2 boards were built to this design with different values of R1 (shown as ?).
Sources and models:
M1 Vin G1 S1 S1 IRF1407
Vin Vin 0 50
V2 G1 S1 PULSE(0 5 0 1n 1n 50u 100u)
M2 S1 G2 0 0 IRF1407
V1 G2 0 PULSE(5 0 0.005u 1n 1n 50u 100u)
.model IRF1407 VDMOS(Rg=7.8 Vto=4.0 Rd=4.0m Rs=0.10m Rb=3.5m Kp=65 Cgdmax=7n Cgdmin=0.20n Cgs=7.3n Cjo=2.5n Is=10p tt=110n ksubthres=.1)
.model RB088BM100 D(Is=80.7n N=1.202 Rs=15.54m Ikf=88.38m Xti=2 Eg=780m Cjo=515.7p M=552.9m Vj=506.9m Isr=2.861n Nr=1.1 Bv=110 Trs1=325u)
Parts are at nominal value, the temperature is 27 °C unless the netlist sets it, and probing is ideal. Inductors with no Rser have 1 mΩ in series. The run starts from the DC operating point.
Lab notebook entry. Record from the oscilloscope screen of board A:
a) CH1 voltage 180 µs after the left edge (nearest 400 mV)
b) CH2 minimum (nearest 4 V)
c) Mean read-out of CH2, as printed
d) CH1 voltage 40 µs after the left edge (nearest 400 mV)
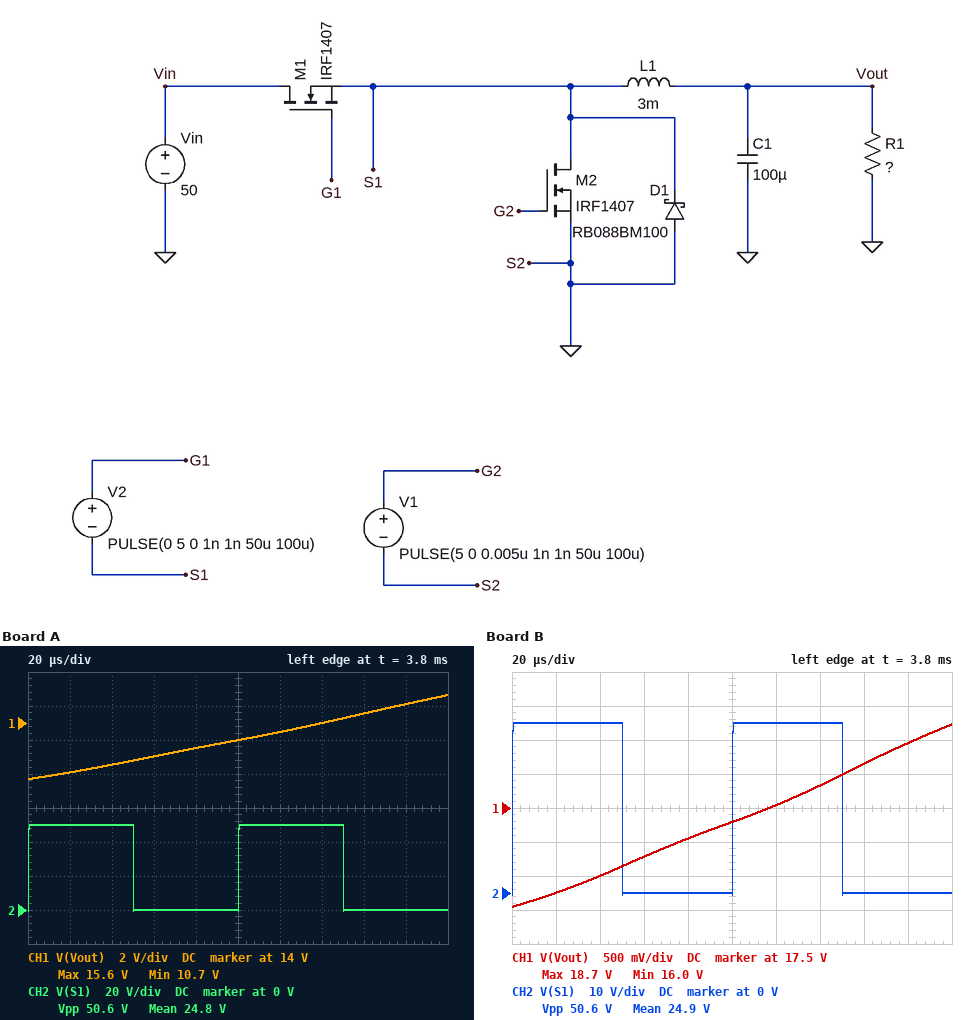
15.2 V
0 V
24.8 V
11.6 V
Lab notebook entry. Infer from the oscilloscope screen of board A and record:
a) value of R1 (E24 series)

62 Ω
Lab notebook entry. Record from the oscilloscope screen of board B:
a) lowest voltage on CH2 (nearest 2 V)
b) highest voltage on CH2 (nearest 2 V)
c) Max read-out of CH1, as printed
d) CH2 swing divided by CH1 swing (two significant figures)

0 V
50 V
18.7 V
19
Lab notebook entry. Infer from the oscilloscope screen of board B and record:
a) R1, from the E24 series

22 Ω
